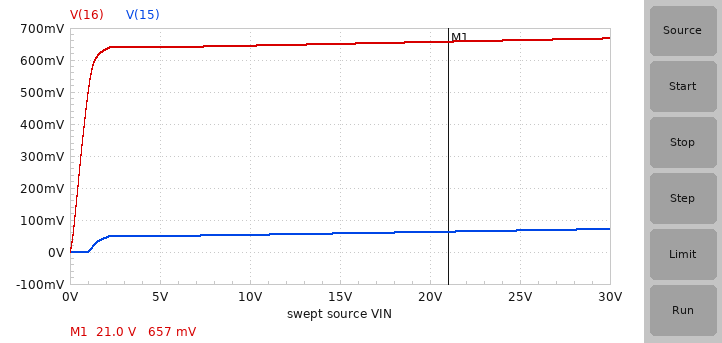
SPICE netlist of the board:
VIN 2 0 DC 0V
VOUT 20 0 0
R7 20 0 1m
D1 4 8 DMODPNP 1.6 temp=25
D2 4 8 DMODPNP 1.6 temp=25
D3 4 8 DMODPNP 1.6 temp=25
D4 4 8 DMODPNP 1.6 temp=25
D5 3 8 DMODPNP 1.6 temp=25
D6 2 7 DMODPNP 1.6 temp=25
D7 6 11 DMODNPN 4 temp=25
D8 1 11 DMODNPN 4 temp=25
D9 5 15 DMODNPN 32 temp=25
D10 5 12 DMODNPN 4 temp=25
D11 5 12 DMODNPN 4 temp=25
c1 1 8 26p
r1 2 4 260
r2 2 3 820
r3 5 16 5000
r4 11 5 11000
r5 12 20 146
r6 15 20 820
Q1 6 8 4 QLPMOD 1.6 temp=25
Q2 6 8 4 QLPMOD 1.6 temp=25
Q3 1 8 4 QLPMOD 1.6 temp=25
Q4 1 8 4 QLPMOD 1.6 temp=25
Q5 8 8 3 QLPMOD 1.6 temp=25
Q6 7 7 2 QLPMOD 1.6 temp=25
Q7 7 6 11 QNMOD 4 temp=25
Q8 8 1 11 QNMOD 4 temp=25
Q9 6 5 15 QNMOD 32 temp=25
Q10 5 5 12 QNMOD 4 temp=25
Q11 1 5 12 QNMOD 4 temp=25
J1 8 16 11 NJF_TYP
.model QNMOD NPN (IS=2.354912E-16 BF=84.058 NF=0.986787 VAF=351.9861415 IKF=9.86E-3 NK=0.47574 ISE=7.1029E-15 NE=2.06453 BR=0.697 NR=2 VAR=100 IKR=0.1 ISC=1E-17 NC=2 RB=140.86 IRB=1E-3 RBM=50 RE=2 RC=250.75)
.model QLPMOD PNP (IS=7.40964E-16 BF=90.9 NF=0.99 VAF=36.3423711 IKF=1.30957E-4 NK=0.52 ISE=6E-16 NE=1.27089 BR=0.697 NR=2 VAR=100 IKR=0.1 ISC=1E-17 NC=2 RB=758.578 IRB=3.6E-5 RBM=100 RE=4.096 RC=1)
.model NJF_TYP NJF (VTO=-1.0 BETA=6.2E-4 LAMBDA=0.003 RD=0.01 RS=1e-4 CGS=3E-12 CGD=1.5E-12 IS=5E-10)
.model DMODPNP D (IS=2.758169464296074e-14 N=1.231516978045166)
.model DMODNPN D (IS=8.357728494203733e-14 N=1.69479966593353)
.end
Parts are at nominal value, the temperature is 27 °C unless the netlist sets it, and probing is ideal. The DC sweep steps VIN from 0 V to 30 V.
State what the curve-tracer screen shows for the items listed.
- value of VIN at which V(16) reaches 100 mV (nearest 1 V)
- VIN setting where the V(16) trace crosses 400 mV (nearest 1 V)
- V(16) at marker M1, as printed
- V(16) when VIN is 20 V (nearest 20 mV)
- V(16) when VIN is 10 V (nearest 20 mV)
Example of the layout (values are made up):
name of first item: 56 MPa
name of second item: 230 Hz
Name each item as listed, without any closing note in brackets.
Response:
value of VIN at which V(16) reaches 100 mV: 0 V
VIN setting where the V(16) trace crosses 400 mV: 1 V
V(16) at marker M1, as printed: 657 mV
V(16) when VIN is 20 V: 660 mV
V(16) when VIN is 10 V: 640 mV
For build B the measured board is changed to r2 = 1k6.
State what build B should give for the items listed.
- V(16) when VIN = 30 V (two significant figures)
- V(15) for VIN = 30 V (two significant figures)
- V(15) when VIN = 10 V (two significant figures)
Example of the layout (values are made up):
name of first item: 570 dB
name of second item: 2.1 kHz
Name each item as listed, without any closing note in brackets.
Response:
V(16) when VIN = 30 V: 680 mV
V(15) for VIN = 30 V: 80 mV
V(15) when VIN = 10 V: 65 mV
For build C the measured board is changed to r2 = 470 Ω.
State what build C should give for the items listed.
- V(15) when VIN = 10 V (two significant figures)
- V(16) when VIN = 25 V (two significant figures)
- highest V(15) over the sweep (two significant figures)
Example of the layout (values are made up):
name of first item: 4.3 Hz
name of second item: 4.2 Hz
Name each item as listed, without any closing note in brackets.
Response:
V(15) when VIN = 10 V: 50 mV
V(16) when VIN = 25 V: 650 mV
highest V(15) over the sweep: 62 mV
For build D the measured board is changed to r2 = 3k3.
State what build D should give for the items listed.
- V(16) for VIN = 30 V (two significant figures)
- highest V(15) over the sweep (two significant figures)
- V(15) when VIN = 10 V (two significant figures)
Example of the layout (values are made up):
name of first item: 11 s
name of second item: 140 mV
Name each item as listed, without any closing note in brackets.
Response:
V(16) for VIN = 30 V: 680 mV
highest V(15) over the sweep: 81 mV
V(15) when VIN = 10 V: 80 mV
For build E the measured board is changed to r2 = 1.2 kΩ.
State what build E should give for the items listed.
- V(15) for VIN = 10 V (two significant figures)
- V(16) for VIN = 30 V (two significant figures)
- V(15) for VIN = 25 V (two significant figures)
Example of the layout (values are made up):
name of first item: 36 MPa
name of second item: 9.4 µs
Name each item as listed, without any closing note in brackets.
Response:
V(15) for VIN = 10 V: 59 mV
V(16) for VIN = 30 V: 680 mV
V(15) for VIN = 25 V: 80 mV
